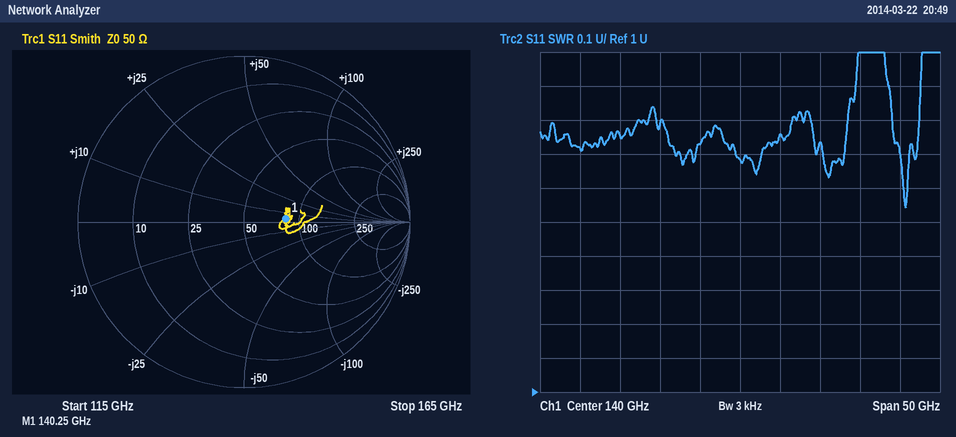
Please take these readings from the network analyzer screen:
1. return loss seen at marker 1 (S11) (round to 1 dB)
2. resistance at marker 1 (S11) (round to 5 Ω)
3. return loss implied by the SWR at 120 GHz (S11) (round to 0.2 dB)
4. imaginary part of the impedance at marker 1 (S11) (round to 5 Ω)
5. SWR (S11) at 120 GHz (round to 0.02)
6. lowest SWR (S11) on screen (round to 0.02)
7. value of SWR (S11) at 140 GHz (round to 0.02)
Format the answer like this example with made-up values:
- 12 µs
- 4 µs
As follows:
- 12 dB
- 85 Ω
- 11.6 dB
- +5 Ω
- 1.72
- 1.54
- 1.68
